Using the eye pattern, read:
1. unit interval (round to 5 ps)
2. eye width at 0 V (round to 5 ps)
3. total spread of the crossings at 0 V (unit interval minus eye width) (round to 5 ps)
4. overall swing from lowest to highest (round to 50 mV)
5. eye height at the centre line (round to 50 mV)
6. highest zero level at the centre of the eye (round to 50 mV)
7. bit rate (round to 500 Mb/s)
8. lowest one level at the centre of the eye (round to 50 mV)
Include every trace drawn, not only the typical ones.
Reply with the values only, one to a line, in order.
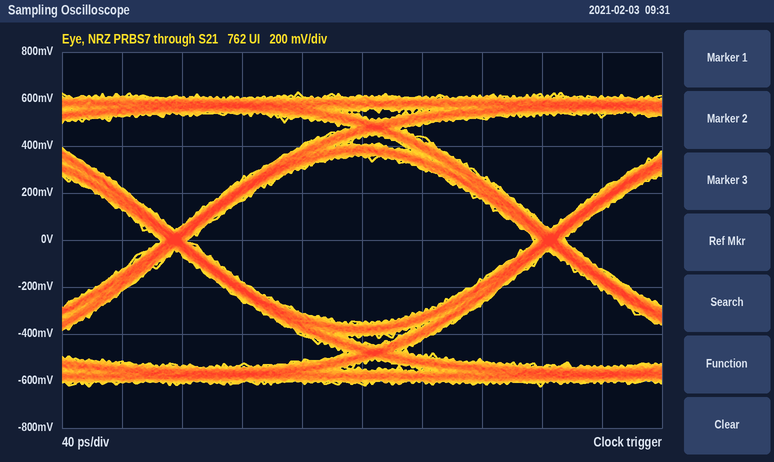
250 ps
230 ps
20 ps
1.25 V
700 mV
-350 mV
4.0 Gb/s
350 mV
